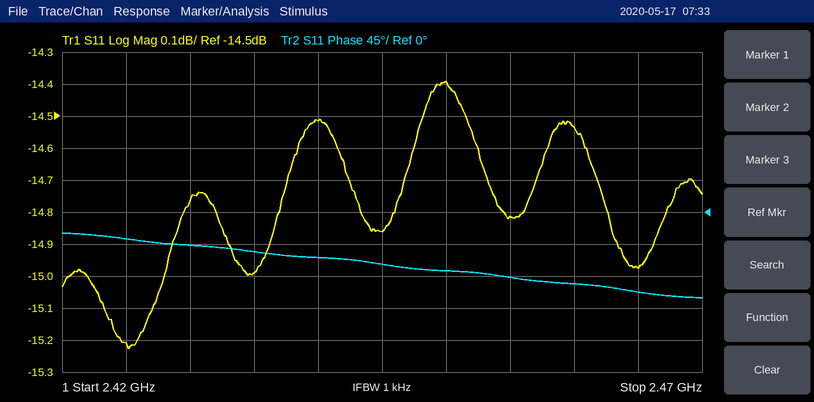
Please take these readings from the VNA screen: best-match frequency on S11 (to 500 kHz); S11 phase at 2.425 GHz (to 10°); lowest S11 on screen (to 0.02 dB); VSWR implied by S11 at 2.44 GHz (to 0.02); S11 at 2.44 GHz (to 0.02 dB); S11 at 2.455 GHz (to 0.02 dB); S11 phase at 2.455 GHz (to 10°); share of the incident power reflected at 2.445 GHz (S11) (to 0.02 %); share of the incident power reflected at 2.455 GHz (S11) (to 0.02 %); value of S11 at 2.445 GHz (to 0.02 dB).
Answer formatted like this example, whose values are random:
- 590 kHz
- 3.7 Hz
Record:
- 2.4250 GHz
- -40°
- -15.22 dB
- 1.46
- -14.52 dB
- -14.82 dB
- -90°
- 3.26 %
- 3.30 %
- -14.86 dB
